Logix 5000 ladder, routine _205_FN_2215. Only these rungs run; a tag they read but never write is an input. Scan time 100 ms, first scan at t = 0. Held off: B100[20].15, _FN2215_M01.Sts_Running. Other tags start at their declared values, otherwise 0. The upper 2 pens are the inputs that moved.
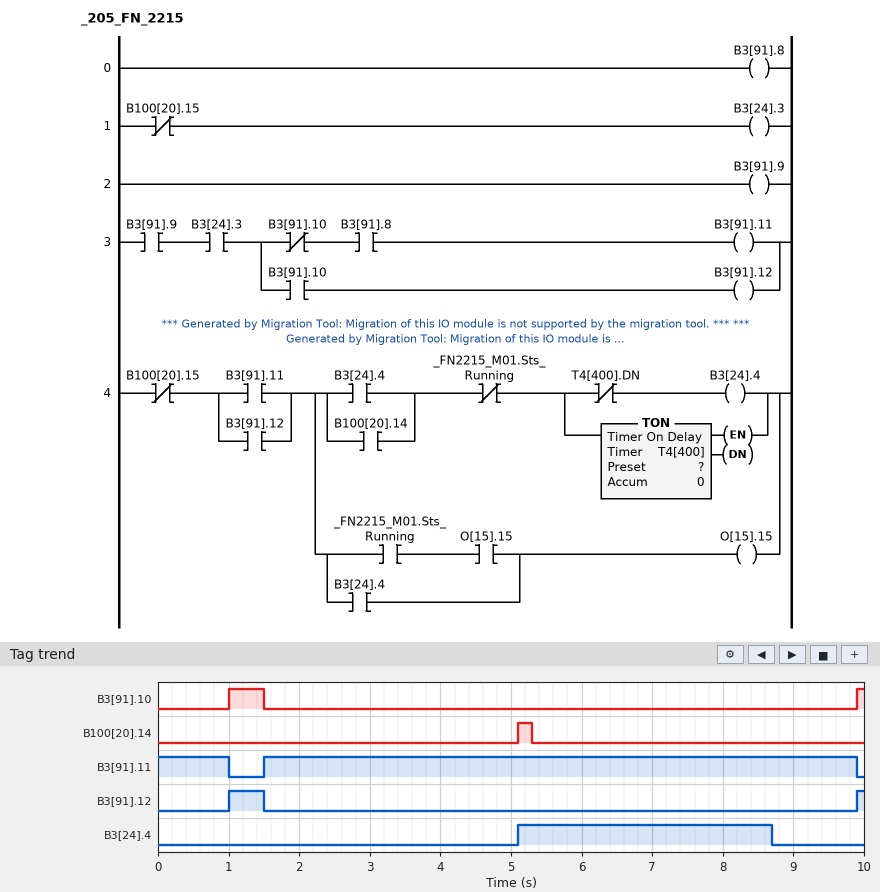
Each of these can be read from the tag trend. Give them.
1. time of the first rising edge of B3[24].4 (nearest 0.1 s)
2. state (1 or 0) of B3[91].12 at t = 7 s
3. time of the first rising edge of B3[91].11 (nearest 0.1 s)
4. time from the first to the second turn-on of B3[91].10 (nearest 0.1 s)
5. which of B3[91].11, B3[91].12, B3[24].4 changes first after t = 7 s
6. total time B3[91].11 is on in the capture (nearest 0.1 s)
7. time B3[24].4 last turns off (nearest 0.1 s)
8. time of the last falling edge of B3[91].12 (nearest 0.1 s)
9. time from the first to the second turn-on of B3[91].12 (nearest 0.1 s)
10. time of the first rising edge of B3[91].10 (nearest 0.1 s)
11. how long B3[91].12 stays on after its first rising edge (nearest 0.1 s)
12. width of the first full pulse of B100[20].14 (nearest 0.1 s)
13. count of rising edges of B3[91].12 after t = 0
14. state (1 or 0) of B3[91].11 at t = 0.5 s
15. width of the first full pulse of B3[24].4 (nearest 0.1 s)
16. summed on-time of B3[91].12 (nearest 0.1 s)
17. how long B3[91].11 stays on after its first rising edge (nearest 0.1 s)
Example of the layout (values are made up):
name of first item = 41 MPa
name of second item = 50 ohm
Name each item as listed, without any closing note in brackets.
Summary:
time of the first rising edge of B3[24].4 = 5.1 s
state (1 or 0) of B3[91].12 at t = 7 s = 0
time of the first rising edge of B3[91].11 = 1.5 s
time from the first to the second turn-on of B3[91].10 = 8.9 s
which of B3[91].11, B3[91].12, B3[24].4 changes first after t = 7 s = B3[24].4
total time B3[91].11 is on in the capture = 9.4 s
time B3[24].4 last turns off = 8.7 s
time of the last falling edge of B3[91].12 = 1.5 s
time from the first to the second turn-on of B3[91].12 = 8.9 s
time of the first rising edge of B3[91].10 = 1.0 s
how long B3[91].12 stays on after its first rising edge = 0.5 s
width of the first full pulse of B100[20].14 = 0.2 s
count of rising edges of B3[91].12 after t = 0 = 2
state (1 or 0) of B3[91].11 at t = 0.5 s = 1
width of the first full pulse of B3[24].4 = 3.6 s
summed on-time of B3[91].12 = 0.6 s
how long B3[91].11 stays on after its first rising edge = 8.4 s
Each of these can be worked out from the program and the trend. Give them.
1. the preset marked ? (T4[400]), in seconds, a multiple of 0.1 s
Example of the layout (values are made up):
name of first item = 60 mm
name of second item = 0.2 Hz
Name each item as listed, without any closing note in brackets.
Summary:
the preset marked ? (T4[400]), in seconds, a multiple of 0.1 s = 3.5 s
